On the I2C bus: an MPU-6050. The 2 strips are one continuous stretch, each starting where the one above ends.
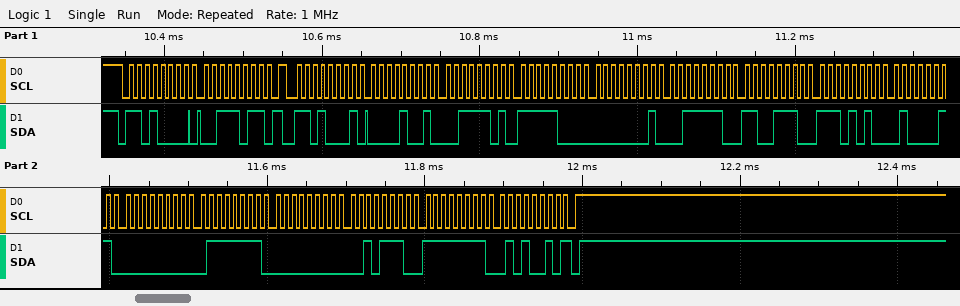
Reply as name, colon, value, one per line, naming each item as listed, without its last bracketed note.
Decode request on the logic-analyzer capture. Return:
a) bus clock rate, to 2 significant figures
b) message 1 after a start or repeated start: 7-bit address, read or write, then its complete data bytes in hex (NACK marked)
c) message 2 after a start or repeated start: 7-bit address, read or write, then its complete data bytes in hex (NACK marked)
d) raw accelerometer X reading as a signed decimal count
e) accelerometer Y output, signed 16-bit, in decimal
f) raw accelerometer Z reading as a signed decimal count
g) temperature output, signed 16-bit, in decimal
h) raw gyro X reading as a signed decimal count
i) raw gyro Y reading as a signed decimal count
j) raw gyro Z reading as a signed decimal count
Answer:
bus clock rate, to 2 significant figures: 100 kHz
message 1 after a start or repeated start: 7-bit address, read or write, then its complete data bytes in hex: 0x68 write: 3B
message 2 after a start or repeated start: 7-bit address, read or write, then its complete data bytes in hex: 0x68 read: 09 3D F8 01 3E CE EA 43 00 7F 00 2E FF 52 NACK
raw accelerometer X reading as a signed decimal count: 2365
accelerometer Y output, signed 16-bit, in decimal: -2047
raw accelerometer Z reading as a signed decimal count: 16078
temperature output, signed 16-bit, in decimal: -5565
raw gyro X reading as a signed decimal count: 127
raw gyro Y reading as a signed decimal count: 46
raw gyro Z reading as a signed decimal count: -174
